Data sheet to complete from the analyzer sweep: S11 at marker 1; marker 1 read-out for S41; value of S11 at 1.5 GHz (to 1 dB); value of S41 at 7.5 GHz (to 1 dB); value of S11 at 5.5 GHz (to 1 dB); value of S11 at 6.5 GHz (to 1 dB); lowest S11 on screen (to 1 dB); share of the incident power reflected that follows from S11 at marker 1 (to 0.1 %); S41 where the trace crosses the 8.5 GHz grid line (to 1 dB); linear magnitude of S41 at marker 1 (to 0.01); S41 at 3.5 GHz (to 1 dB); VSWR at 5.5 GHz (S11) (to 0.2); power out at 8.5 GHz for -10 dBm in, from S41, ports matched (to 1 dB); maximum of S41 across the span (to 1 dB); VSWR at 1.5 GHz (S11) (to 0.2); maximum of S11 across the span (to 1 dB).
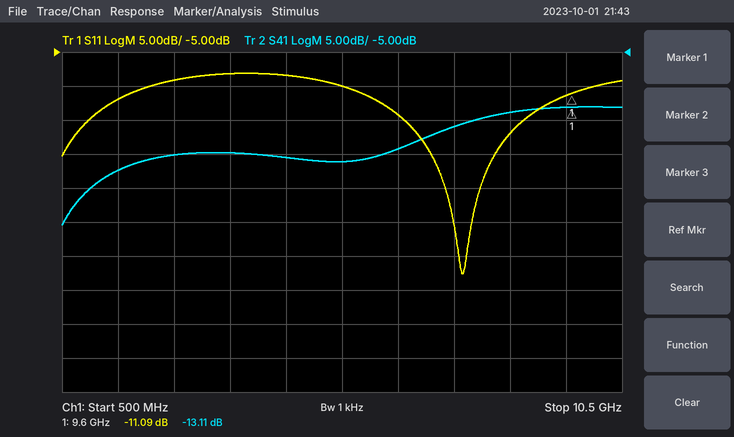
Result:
-11.09 dB
-13.11 dB
-12 dB
-16 dB
-10 dB
-14 dB
-38 dB
7.8 %
-14 dB
0.22
-20 dB
2.0
-24 dBm
-13 dB
1.6
-8 dB
